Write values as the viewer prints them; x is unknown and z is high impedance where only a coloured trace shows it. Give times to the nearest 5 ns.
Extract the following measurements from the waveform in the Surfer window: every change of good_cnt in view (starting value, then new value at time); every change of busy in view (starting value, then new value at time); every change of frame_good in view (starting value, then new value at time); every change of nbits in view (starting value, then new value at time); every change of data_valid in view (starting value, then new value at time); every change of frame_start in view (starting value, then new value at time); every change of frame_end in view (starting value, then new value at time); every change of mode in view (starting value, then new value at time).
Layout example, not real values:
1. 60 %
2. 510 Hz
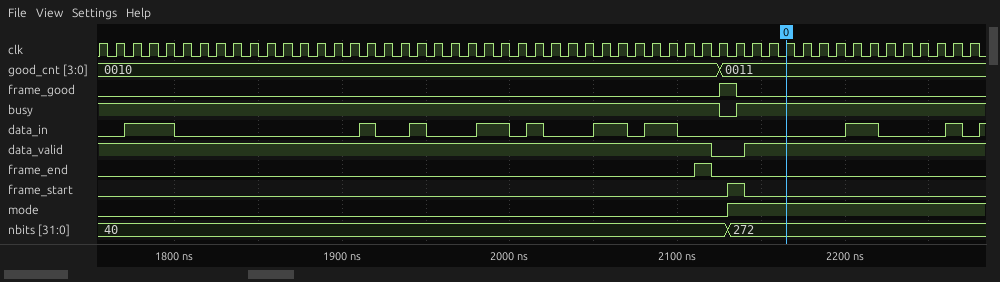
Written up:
1. 0010, 0011 at 2125 ns
2. 1, 0 at 2125 ns, 1 at 2135 ns
3. 0, 1 at 2125 ns, 0 at 2135 ns
4. 40, 272 at 2130 ns
5. 1, 0 at 2120 ns, 1 at 2140 ns
6. 0, 1 at 2130 ns, 0 at 2140 ns
7. 0, 1 at 2110 ns, 0 at 2120 ns
8. 0, 1 at 2130 ns
